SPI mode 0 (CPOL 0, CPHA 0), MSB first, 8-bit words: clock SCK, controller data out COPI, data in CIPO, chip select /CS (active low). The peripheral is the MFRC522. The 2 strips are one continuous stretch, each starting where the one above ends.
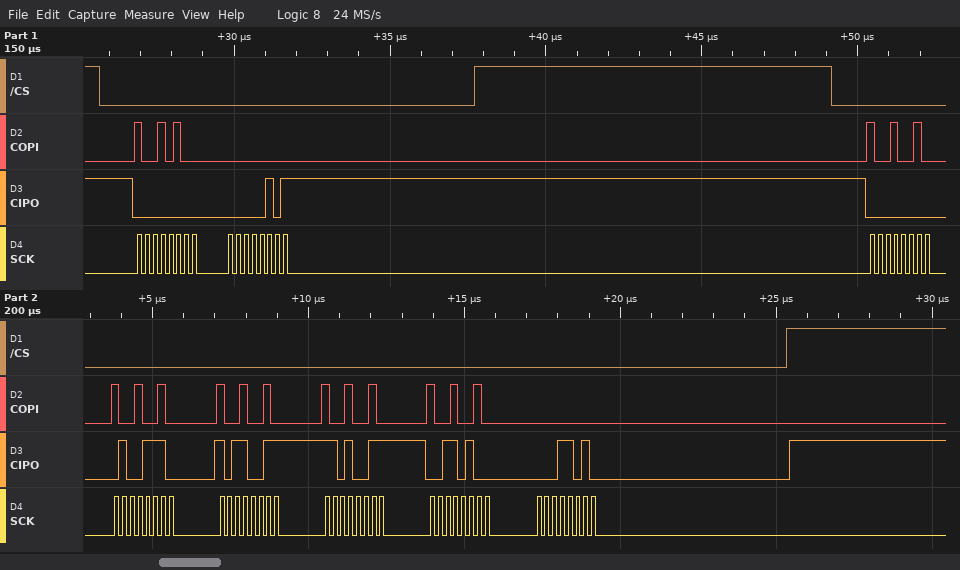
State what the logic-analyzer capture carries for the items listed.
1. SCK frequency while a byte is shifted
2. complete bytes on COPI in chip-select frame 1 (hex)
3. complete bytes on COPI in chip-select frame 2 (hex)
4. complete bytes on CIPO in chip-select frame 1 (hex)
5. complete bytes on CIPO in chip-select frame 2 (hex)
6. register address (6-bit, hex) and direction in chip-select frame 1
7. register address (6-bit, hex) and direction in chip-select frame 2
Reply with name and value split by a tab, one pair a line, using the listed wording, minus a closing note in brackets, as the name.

SCK frequency while a byte is shifted	4 MHz
complete bytes on COPI in chip-select frame 1	94 00
complete bytes on COPI in chip-select frame 2	92 92 92 92 92 00
complete bytes on CIPO in chip-select frame 1	00 05
complete bytes on CIPO in chip-select frame 2	00 4E B3 D3 34 1A
register address (6-bit, hex) and direction in chip-select frame 1	0x0A read
register address (6-bit, hex) and direction in chip-select frame 2	0x09 read
